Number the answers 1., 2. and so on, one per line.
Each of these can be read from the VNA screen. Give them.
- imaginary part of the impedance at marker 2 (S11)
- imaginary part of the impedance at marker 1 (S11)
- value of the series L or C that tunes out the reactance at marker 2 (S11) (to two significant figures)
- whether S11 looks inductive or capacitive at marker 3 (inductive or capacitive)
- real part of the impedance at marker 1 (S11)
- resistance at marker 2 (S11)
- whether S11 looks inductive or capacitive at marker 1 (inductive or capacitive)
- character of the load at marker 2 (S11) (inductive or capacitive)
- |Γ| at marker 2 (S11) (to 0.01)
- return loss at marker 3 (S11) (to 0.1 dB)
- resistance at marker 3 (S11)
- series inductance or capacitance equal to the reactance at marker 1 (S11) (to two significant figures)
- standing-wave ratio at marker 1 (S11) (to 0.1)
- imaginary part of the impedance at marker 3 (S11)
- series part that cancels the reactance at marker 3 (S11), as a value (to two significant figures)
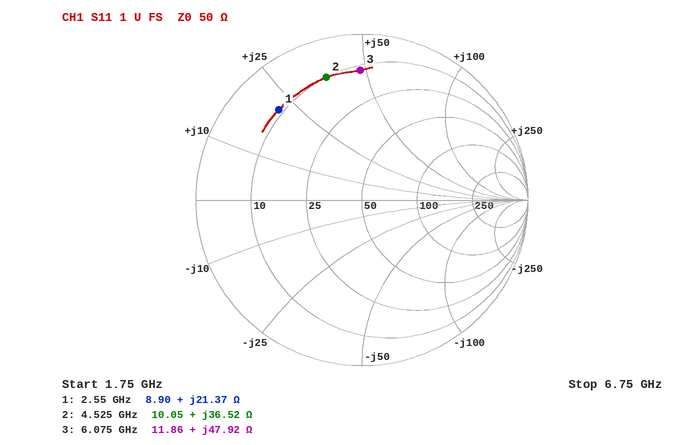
1. +36.52 Ω
2. +21.37 Ω
3. 960 fF
4. inductive
5. 8.90 Ω
6. 10.05 Ω
7. inductive
8. inductive
9. 0.77
10. 2.1 dB
11. 11.86 Ω
12. 1.3 nH
13. 6.7
14. +47.92 Ω
15. 550 fF
